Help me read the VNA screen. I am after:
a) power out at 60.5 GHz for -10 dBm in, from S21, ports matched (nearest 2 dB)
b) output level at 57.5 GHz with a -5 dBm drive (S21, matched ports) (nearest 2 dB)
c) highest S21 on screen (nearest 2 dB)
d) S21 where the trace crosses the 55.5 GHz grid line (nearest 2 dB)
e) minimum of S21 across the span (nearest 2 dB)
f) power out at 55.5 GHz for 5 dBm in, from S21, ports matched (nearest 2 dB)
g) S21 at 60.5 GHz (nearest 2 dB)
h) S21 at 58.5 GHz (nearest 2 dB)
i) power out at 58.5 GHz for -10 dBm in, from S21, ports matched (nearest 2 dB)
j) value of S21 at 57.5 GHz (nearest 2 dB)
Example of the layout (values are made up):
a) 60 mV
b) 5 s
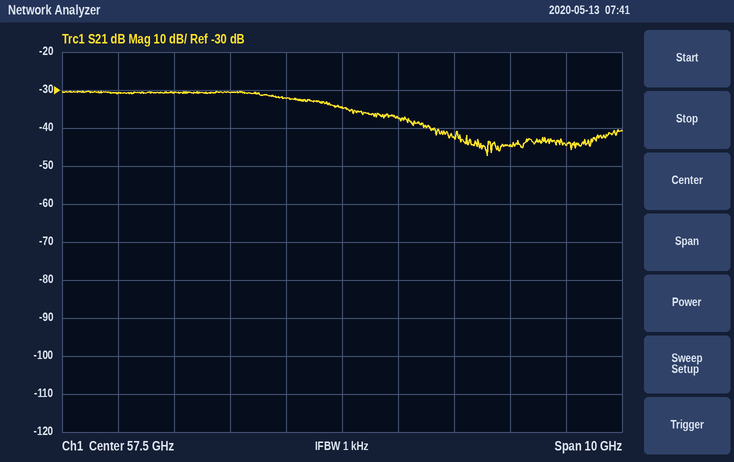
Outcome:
a) -54 dBm
b) -40 dBm
c) -30 dB
d) -30 dB
e) -48 dB
f) -26 dBm
g) -44 dB
h) -38 dB
i) -48 dBm
j) -34 dB
